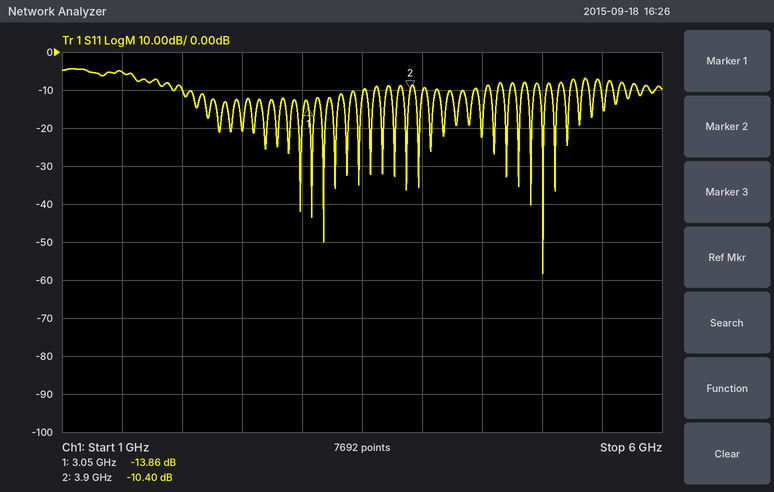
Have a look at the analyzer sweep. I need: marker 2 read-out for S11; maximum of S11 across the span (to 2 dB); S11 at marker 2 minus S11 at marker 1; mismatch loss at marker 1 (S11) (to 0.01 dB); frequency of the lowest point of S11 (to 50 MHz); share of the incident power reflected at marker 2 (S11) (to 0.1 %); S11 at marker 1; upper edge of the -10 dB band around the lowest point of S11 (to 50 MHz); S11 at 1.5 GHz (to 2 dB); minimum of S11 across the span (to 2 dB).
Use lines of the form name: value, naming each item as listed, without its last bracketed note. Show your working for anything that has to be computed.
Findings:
marker 2 read-out for S11: -10.40 dB
maximum of S11 across the span: -4 dB
S11 at marker 2 minus S11 at marker 1: -10.4 − (-13.86) = 3.46 dB
mismatch loss at marker 1 (S11): −10 log10(1 − 10^(-13.86/10)) ≈ 0.18 dB
frequency of the lowest point of S11: 5.00 GHz
share of the incident power reflected at marker 2 (S11): 10^(-10.4/10) ≈ 9.1 %
S11 at marker 1: -13.86 dB
upper edge of the -10 dB band around the lowest point of S11: 5.05 GHz
S11 at 1.5 GHz: -6 dB
minimum of S11 across the span: -58 dB
